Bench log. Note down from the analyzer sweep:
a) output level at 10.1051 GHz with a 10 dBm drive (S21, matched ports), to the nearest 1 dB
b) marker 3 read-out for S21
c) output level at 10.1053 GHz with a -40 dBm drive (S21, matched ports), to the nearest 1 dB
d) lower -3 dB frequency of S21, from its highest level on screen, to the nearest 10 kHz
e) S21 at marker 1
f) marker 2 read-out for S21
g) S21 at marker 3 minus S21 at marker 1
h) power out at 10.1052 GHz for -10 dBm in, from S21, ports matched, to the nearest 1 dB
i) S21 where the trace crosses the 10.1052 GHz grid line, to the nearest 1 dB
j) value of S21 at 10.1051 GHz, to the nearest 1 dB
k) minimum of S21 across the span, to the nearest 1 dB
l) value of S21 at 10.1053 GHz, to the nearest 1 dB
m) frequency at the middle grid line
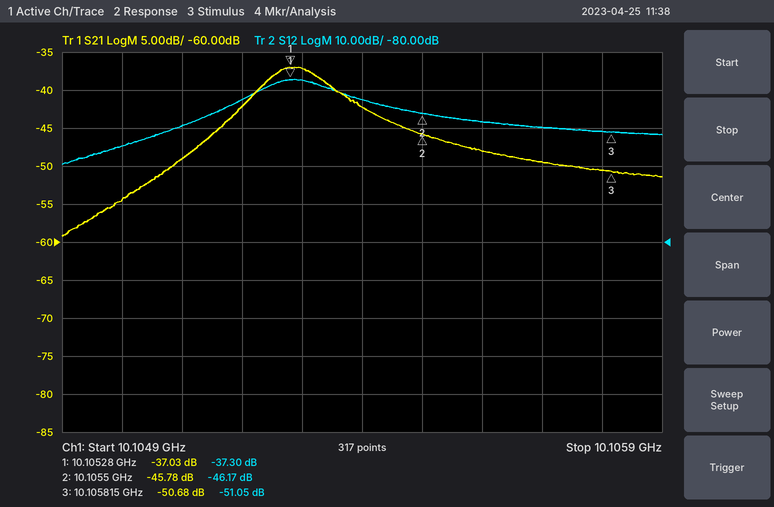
-39 dBm
-50.68 dB
-77 dBm
10.10523 GHz
-37.03 dB
-45.78 dB
-13.65 dB
-52 dBm
-42 dB
-49 dB
-59 dB
-37 dB
10.1054 GHz
